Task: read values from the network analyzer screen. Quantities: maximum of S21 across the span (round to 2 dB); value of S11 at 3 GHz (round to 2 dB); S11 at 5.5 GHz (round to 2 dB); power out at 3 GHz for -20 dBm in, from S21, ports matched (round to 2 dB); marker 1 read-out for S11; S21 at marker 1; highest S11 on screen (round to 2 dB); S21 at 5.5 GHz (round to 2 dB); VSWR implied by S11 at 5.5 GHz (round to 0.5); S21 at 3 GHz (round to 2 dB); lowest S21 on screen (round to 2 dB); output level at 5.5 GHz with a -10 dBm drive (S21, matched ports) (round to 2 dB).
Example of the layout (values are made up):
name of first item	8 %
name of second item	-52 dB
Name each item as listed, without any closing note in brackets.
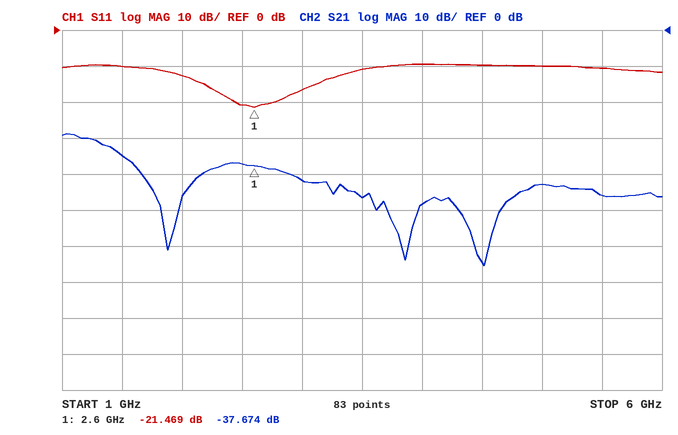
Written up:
maximum of S21 across the span	-28 dB
value of S11 at 3 GHz	-16 dB
S11 at 5.5 GHz	-10 dB
power out at 3 GHz for -20 dBm in, from S21, ports matched	-62 dBm
marker 1 read-out for S11	-21.469 dB
S21 at marker 1	-37.674 dB
highest S11 on screen	-10 dB
S21 at 5.5 GHz	-46 dB
VSWR implied by S11 at 5.5 GHz	2.0
S21 at 3 GHz	-42 dB
lowest S21 on screen	-66 dB
output level at 5.5 GHz with a -10 dBm drive (S21, matched ports)	-56 dBm
